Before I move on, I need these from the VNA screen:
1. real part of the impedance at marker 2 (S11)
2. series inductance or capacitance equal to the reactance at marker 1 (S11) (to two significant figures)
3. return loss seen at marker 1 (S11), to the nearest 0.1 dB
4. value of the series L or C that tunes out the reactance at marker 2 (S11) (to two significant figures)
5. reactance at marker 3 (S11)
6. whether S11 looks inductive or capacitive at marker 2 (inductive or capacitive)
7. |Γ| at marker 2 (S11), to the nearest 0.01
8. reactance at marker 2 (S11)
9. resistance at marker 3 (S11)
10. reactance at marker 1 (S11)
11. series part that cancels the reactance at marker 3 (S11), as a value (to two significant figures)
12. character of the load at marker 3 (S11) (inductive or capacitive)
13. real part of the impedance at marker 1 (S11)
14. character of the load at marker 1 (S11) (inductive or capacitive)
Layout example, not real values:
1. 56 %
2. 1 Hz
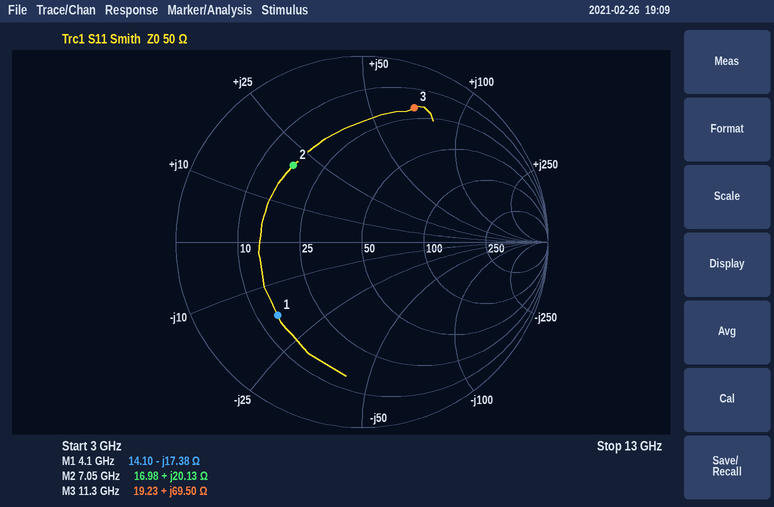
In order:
1. 16.98 Ω
2. 2.2 pF
3. 4.4 dB
4. 1.1 pF
5. +69.50 Ω
6. inductive
7. 0.55
8. +20.13 Ω
9. 19.23 Ω
10. -17.38 Ω
11. 200 fF
12. inductive
13. 14.10 Ω
14. capacitive
